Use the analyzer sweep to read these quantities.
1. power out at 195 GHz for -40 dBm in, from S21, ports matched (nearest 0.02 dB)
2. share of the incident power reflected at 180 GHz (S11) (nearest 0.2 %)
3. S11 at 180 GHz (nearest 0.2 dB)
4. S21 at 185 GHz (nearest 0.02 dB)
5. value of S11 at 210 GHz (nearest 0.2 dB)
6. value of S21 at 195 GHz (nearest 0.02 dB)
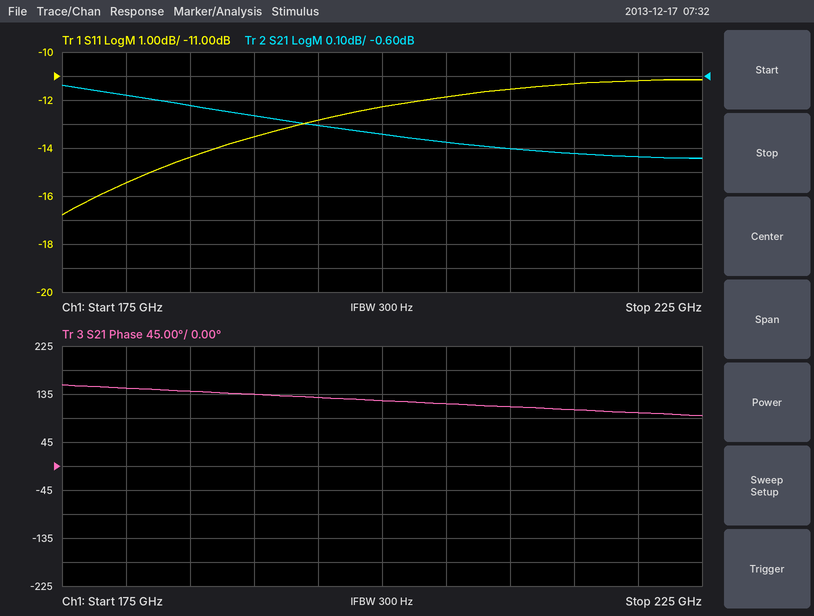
-40.80 dBm
2.8 %
-15.4 dB
-0.72 dB
-11.6 dB
-0.80 dB
